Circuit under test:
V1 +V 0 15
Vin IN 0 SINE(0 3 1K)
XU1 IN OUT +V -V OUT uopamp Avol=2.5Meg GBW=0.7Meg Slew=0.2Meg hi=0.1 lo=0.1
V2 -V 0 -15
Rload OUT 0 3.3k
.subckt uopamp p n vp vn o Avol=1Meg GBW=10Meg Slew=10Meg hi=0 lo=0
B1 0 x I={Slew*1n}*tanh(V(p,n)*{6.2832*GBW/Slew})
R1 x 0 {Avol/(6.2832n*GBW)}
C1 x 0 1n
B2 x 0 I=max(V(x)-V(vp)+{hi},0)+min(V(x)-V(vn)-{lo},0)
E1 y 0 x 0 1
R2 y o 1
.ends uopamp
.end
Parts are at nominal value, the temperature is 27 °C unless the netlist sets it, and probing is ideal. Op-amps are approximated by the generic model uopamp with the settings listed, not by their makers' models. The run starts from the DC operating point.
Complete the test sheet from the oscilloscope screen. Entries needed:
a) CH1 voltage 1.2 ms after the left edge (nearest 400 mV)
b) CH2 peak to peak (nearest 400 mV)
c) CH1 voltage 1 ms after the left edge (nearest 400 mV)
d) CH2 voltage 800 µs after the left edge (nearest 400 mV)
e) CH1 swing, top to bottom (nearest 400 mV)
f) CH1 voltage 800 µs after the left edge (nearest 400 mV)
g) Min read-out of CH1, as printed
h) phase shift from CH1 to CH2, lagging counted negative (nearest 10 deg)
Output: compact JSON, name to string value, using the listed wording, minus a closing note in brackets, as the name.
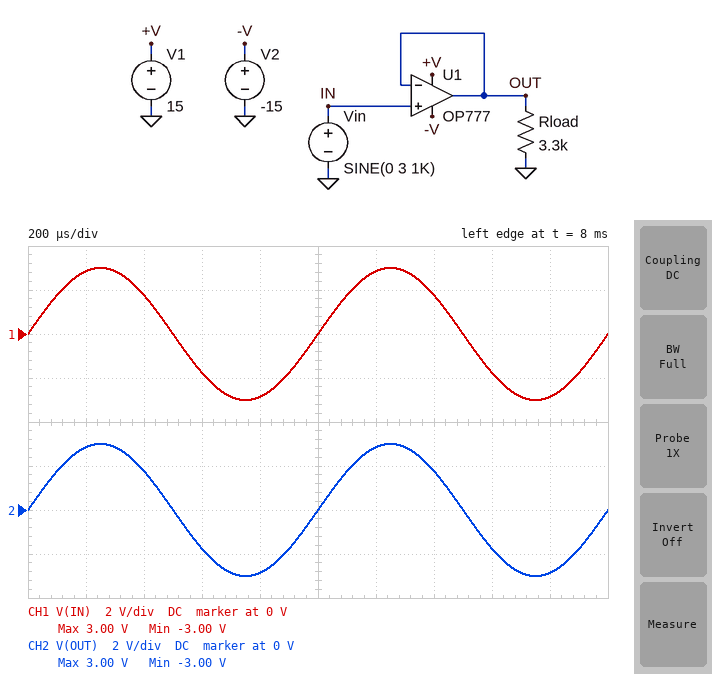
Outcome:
{"CH1 voltage 1.2 ms after the left edge": "2.8 V", "CH2 peak to peak": "6.0 V", "CH1 voltage 1 ms after the left edge": "0 V", "CH2 voltage 800 µs after the left edge": "-2.8 V", "CH1 swing, top to bottom": "6.0 V", "CH1 voltage 800 µs after the left edge": "-2.8 V", "Min read-out of CH1, as printed": "-3.00 V", "phase shift from CH1 to CH2, lagging counted negative": "0 deg"}
